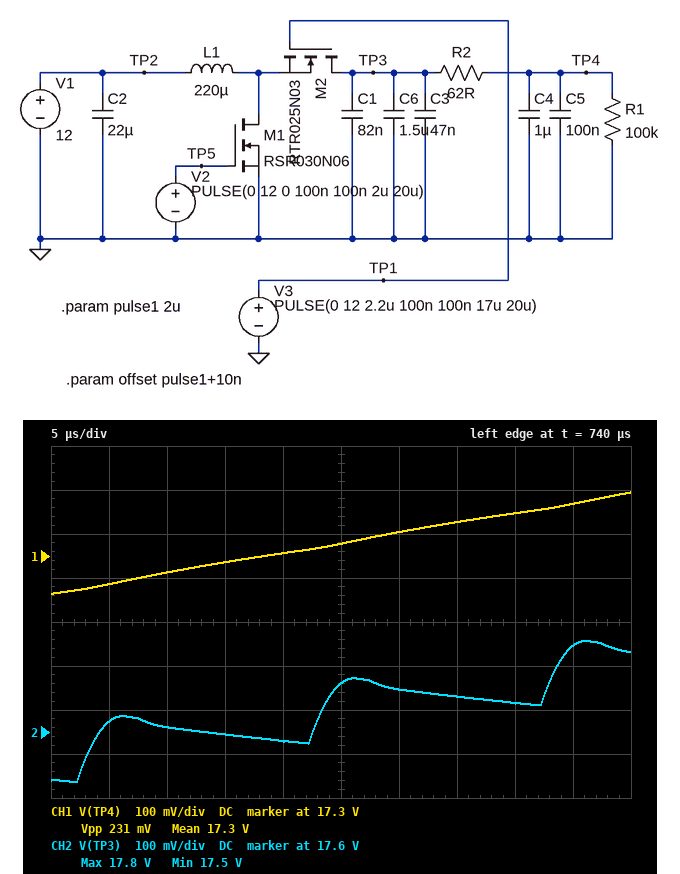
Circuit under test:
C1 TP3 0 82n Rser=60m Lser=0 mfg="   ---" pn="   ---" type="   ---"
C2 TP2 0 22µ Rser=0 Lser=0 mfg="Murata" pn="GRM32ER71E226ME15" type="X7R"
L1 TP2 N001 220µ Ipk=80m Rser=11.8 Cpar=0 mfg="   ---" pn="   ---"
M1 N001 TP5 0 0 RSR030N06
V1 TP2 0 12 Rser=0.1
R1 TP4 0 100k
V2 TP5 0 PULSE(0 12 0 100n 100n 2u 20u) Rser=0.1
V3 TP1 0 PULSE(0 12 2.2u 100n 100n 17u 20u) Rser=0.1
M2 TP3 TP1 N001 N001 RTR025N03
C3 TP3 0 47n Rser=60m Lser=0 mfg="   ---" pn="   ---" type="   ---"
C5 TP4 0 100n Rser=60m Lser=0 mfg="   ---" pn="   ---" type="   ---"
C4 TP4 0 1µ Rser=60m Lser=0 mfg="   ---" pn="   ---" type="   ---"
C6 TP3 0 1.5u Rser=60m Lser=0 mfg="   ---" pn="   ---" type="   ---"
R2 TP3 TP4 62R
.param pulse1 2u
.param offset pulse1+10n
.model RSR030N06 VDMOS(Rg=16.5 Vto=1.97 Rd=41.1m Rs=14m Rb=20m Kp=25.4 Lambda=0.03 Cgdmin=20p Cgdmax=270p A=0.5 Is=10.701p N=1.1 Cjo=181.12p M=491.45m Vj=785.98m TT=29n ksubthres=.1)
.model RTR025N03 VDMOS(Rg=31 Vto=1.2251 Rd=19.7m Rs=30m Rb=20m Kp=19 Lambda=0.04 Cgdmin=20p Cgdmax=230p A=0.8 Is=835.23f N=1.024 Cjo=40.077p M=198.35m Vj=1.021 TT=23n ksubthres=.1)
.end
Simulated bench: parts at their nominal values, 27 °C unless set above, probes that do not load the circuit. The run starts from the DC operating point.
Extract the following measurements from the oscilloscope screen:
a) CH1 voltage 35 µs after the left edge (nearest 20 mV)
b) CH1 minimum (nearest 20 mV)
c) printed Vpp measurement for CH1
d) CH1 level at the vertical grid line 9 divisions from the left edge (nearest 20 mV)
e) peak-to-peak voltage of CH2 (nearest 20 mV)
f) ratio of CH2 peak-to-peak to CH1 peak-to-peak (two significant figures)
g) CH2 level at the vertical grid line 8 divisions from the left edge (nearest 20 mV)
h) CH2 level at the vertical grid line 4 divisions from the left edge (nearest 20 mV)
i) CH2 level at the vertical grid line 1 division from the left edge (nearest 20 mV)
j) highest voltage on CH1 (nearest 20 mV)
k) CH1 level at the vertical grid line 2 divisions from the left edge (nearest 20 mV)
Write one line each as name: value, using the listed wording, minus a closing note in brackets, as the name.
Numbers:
CH1 voltage 35 µs after the left edge: 17.38 V
CH1 minimum: 17.22 V
printed Vpp measurement for CH1: 231 mV
CH1 level at the vertical grid line 9 divisions from the left edge: 17.42 V
peak-to-peak voltage of CH2: 320 mV
ratio of CH2 peak-to-peak to CH1 peak-to-peak: 1.4
CH2 level at the vertical grid line 8 divisions from the left edge: 17.66 V
CH2 level at the vertical grid line 4 divisions from the left edge: 17.58 V
CH2 level at the vertical grid line 1 division from the left edge: 17.62 V
highest voltage on CH1: 17.44 V
CH1 level at the vertical grid line 2 divisions from the left edge: 17.26 V
